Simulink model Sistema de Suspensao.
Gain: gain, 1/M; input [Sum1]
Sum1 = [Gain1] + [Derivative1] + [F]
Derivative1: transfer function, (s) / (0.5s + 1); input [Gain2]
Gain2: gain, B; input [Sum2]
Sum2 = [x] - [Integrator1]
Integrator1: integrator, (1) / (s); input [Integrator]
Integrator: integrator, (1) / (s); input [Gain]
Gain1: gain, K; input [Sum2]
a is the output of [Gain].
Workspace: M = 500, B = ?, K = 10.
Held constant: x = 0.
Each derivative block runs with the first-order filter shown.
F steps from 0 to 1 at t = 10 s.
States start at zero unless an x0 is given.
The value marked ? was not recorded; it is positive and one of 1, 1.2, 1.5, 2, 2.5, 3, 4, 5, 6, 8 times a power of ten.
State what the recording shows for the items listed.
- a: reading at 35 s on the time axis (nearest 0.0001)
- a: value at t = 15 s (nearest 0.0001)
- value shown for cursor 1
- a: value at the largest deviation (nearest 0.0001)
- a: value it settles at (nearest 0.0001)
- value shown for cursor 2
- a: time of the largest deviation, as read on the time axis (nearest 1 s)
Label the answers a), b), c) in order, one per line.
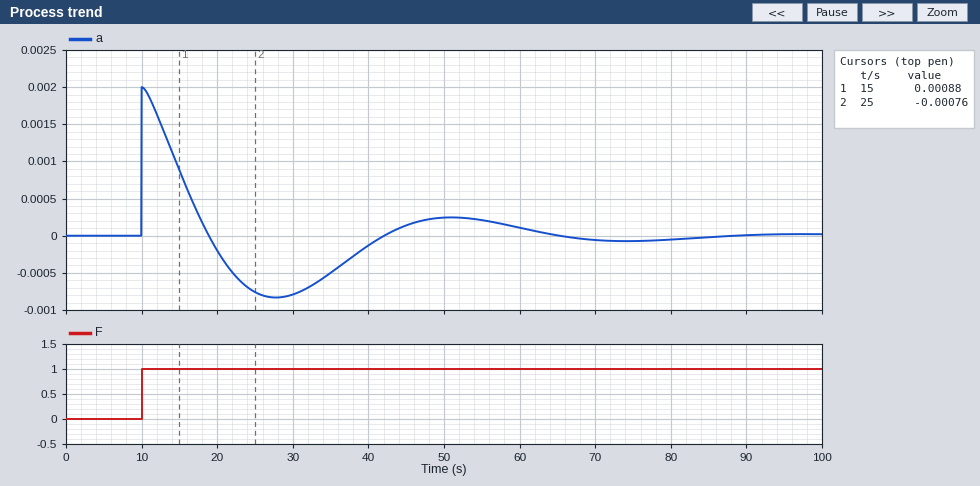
a) -0.0005
b) 0.0009
c) 0.00088
d) 0.0020
e) 0.0000
f) -0.00076
g) 10 s
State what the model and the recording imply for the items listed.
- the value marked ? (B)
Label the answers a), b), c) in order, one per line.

a) 50
